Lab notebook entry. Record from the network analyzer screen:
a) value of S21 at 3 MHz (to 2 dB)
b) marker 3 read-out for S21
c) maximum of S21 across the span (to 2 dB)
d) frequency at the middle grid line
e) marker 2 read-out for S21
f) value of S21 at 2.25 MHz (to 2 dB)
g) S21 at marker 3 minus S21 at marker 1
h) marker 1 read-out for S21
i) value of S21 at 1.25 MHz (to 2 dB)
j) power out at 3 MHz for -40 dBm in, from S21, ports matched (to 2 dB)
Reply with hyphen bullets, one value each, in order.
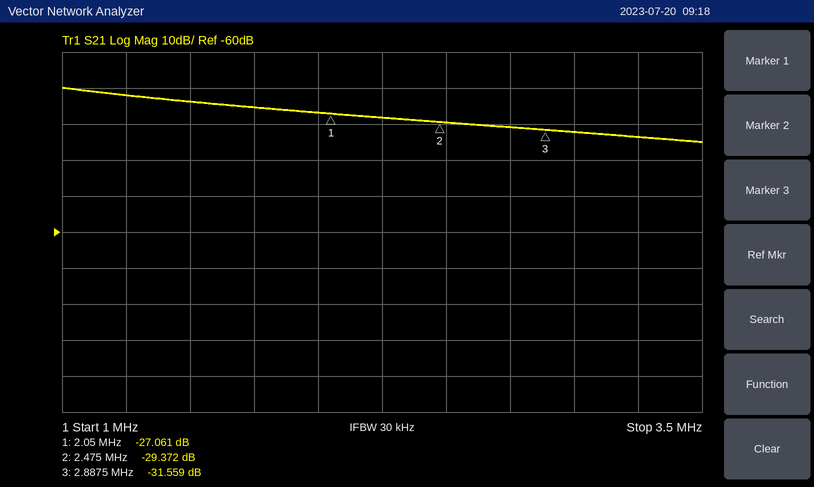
- -32 dB
- -31.559 dB
- -20 dB
- 2.25 MHz
- -29.372 dB
- -28 dB
- -4.498 dB
- -27.061 dB
- -22 dB
- -72 dBm
